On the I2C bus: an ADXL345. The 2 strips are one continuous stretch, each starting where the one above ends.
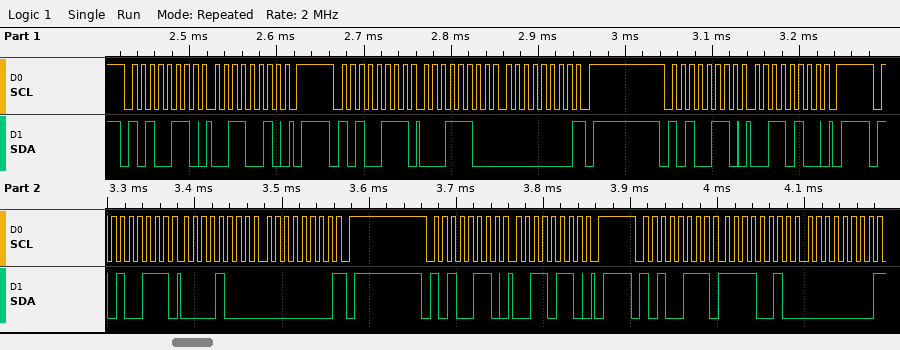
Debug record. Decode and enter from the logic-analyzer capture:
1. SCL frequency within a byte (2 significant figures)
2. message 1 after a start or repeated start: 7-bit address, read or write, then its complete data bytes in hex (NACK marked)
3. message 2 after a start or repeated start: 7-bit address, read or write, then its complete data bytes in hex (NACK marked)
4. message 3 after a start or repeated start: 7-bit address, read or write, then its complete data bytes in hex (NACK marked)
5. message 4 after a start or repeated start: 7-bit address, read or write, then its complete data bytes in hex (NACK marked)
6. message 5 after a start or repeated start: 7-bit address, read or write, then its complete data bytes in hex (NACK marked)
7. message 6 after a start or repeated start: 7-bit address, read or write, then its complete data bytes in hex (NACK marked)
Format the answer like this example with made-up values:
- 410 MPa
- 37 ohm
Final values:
- 100 kHz
- 0x53 write: 32
- 0x53 read: 1C 00 NACK
- 0x53 write: 34
- 0x53 read: 08 00 NACK
- 0x53 write: 36
- 0x53 read: F2 00 NACK
